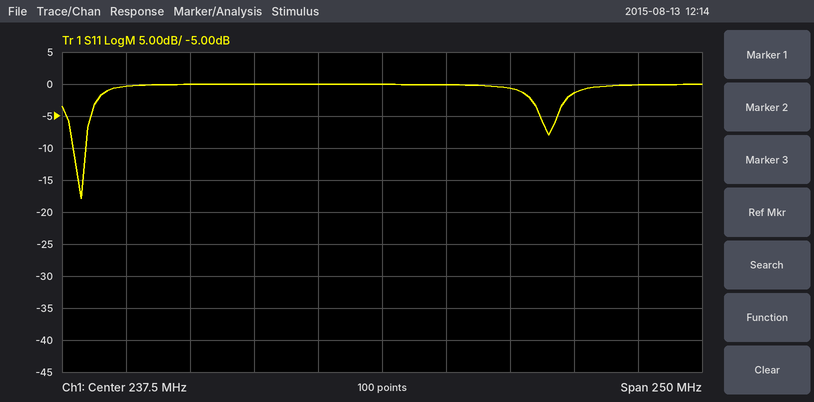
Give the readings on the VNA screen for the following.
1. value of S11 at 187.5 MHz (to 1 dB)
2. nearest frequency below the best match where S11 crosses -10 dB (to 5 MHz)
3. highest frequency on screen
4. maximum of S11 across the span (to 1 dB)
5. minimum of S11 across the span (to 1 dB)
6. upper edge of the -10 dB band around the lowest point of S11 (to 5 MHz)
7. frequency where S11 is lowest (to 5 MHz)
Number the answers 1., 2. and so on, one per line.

1. 0 dB
2. 115 MHz
3. 362.5 MHz
4. 0 dB
5. -18 dB
6. 120 MHz
7. 120 MHz
